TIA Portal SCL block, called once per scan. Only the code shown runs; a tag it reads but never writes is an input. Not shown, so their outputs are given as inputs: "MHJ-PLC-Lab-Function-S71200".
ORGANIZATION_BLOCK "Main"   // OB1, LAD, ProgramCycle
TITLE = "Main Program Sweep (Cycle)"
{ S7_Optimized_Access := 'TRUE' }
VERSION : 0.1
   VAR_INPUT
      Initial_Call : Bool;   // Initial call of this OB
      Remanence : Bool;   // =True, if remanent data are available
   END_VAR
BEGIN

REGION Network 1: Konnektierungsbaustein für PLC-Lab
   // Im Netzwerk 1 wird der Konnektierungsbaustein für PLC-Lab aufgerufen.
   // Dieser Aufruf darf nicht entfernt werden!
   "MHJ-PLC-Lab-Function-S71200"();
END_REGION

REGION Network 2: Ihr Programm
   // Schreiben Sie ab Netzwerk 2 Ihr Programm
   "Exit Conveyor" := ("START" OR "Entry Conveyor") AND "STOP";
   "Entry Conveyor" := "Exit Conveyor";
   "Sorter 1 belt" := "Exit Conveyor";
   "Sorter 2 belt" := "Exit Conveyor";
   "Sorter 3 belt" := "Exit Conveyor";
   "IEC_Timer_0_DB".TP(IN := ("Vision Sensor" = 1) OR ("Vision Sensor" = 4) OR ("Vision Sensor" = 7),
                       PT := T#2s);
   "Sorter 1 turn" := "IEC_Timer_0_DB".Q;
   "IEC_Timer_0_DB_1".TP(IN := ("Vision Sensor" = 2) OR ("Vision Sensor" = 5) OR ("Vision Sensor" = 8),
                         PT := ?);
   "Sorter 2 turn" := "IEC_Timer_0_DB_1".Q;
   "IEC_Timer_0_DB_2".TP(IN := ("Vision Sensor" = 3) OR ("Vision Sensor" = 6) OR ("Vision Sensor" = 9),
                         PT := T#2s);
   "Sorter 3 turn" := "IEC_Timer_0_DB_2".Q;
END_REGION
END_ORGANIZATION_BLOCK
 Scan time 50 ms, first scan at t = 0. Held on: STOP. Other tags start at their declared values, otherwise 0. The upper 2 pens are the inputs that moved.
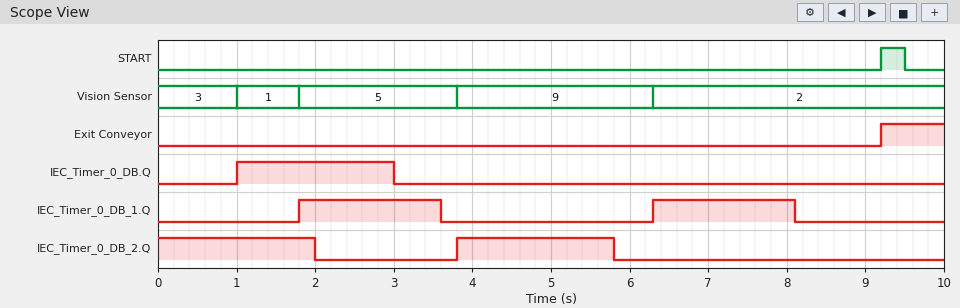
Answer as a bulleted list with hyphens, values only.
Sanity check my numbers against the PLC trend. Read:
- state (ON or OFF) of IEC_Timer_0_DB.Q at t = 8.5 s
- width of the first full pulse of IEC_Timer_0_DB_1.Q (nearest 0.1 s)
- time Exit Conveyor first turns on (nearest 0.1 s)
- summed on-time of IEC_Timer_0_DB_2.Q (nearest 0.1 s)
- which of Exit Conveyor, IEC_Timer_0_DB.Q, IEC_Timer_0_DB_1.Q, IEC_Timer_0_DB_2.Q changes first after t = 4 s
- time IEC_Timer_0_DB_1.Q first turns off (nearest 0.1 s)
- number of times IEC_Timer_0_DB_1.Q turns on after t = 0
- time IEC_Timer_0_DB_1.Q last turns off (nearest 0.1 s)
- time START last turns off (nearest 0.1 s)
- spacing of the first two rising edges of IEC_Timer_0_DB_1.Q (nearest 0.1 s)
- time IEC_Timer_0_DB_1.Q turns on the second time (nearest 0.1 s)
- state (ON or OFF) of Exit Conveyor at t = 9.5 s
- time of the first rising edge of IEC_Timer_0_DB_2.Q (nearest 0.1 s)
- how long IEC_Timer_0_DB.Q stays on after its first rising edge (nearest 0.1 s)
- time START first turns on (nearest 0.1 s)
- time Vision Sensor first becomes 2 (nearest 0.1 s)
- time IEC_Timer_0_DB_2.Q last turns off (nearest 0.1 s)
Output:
- OFF
- 1.8 s
- 9.2 s
- 4.0 s
- IEC_Timer_0_DB_2.Q
- 3.6 s
- 2
- 8.1 s
- 9.5 s
- 4.5 s
- 6.3 s
- ON
- 3.8 s
- 2.0 s
- 9.2 s
- 6.3 s
- 5.8 s
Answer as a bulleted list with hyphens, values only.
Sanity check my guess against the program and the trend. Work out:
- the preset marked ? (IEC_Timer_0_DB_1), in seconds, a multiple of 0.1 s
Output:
- 1.8 s
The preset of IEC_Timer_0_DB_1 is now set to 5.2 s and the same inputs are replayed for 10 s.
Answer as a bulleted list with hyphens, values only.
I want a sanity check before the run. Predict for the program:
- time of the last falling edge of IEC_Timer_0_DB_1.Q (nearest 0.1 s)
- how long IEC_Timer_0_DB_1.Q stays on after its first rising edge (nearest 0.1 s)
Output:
- 7.0 s
- 5.2 s
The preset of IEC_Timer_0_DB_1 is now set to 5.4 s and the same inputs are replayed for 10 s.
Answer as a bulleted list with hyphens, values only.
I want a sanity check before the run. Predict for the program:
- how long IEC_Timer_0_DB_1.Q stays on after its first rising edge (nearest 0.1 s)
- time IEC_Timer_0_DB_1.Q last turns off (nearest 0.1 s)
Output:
- 5.4 s
- 7.2 s
